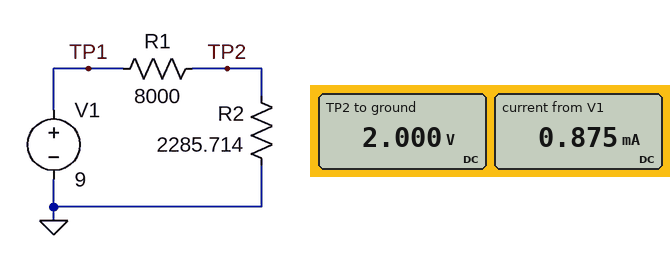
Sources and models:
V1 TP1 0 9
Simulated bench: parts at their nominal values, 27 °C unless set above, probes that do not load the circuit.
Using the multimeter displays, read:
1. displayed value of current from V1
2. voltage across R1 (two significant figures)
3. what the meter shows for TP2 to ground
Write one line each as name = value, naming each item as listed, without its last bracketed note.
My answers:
displayed value of current from V1 = 0.875 mA
voltage across R1 = 7.0 V
what the meter shows for TP2 to ground = 2.000 V
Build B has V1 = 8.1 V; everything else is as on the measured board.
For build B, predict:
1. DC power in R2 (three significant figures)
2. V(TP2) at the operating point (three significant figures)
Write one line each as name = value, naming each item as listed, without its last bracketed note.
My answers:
DC power in R2 = 1.42 mW
V(TP2) at the operating point = 1.80 V
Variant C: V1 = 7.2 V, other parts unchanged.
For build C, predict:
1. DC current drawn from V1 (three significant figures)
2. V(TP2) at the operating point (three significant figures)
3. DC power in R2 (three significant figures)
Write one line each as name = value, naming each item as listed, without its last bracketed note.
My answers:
DC current drawn from V1 = 700 µA
V(TP2) at the operating point = 1.60 V
DC power in R2 = 1.12 mW
